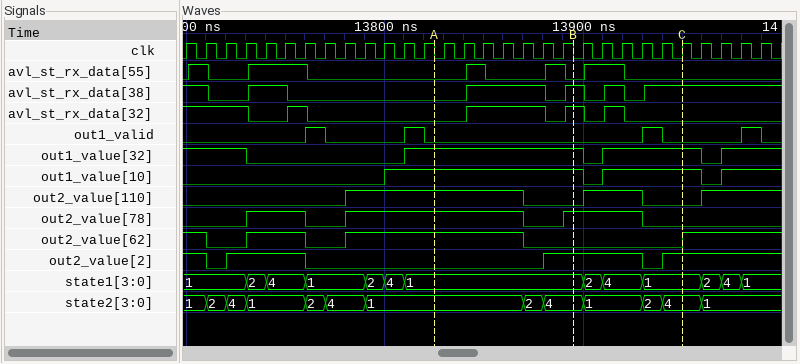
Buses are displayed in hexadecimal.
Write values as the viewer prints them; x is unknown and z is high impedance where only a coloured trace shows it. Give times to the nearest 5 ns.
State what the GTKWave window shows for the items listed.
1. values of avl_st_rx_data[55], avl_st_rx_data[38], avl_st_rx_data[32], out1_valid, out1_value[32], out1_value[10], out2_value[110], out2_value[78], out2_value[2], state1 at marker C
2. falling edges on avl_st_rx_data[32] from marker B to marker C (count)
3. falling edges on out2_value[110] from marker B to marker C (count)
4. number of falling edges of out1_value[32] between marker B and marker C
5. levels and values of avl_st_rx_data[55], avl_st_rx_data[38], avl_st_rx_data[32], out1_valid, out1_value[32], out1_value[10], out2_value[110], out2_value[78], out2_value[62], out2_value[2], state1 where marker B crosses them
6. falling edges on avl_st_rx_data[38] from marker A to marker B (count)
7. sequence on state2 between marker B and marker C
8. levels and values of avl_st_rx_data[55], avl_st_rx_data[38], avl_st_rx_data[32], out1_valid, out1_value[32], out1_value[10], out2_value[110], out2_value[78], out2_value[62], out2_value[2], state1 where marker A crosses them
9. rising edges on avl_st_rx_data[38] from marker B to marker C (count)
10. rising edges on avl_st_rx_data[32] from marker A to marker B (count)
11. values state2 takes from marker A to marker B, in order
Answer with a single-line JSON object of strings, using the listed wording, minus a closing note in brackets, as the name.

{"values of avl_st_rx_data[55], avl_st_rx_data[38], avl_st_rx_data[32], out1_valid, out1_value[32], out1_value[10], out2_value[110], out2_value[78], out2_value[2], state1 at marker C": "avl_st_rx_data[55]=0, avl_st_rx_data[38]=1, avl_st_rx_data[32]=0, out1_valid=0, out1_value[32]=1, out1_value[10]=1, out2_value[110]=0, out2_value[78]=0, out2_value[2]=1, state1=1", "falling edges on avl_st_rx_data[32] from marker B to marker C": "2", "falling edges on out2_value[110] from marker B to marker C": "1", "number of falling edges of out1_value[32] between marker B and marker C": "1", "levels and values of avl_st_rx_data[55], avl_st_rx_data[38], avl_st_rx_data[32], out1_valid, out1_value[32], out1_value[10], out2_value[110], out2_value[78], out2_value[62], out2_value[2], state1 where marker B crosses them": "avl_st_rx_data[55]=0, avl_st_rx_data[38]=1, avl_st_rx_data[32]=1, out1_valid=0, out1_value[32]=1, out1_value[10]=1, out2_value[110]=0, out2_value[78]=1, out2_value[62]=0, out2_value[2]=1, state1=1", "falling edges on avl_st_rx_data[38] from marker A to marker B": "1", "sequence on state2 between marker B and marker C": "4, 1, 2, 4", "levels and values of avl_st_rx_data[55], avl_st_rx_data[38], avl_st_rx_data[32], out1_valid, out1_value[32], out1_value[10], out2_value[110], out2_value[78], out2_value[62], out2_value[2], state1 where marker A crosses them": "avl_st_rx_data[55]=0, avl_st_rx_data[38]=0, avl_st_rx_data[32]=0, out1_valid=0, out1_value[32]=1, out1_value[10]=1, out2_value[110]=1, out2_value[78]=1, out2_value[62]=1, out2_value[2]=0, state1=1", "rising edges on avl_st_rx_data[38] from marker B to marker C": "2", "rising edges on avl_st_rx_data[32] from marker A to marker B": "2", "values state2 takes from marker A to marker B, in order": "1, 2, 4"}
